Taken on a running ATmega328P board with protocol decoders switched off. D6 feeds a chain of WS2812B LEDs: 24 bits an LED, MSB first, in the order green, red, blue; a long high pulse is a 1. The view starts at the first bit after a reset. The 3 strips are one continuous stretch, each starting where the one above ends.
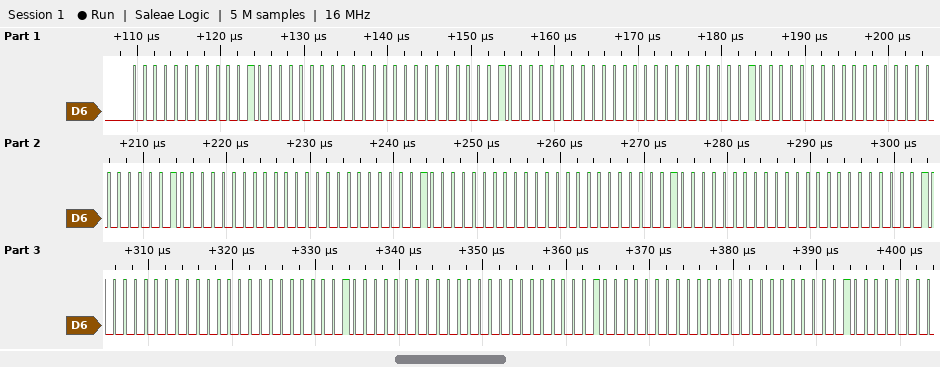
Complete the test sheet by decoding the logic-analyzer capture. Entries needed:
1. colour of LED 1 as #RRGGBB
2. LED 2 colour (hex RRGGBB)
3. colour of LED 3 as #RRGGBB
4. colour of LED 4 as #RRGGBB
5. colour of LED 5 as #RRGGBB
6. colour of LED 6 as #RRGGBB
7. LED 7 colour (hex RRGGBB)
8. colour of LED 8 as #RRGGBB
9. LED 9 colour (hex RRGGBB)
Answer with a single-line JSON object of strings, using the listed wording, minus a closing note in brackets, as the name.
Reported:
{"colour of LED 1 as #RRGGBB": "#100000", "LED 2 colour": "#100000", "colour of LED 3 as #RRGGBB": "#100000", "colour of LED 4 as #RRGGBB": "#100000", "colour of LED 5 as #RRGGBB": "#100000", "colour of LED 6 as #RRGGBB": "#100000", "LED 7 colour": "#100000", "colour of LED 8 as #RRGGBB": "#100000", "LED 9 colour": "#100000"}
